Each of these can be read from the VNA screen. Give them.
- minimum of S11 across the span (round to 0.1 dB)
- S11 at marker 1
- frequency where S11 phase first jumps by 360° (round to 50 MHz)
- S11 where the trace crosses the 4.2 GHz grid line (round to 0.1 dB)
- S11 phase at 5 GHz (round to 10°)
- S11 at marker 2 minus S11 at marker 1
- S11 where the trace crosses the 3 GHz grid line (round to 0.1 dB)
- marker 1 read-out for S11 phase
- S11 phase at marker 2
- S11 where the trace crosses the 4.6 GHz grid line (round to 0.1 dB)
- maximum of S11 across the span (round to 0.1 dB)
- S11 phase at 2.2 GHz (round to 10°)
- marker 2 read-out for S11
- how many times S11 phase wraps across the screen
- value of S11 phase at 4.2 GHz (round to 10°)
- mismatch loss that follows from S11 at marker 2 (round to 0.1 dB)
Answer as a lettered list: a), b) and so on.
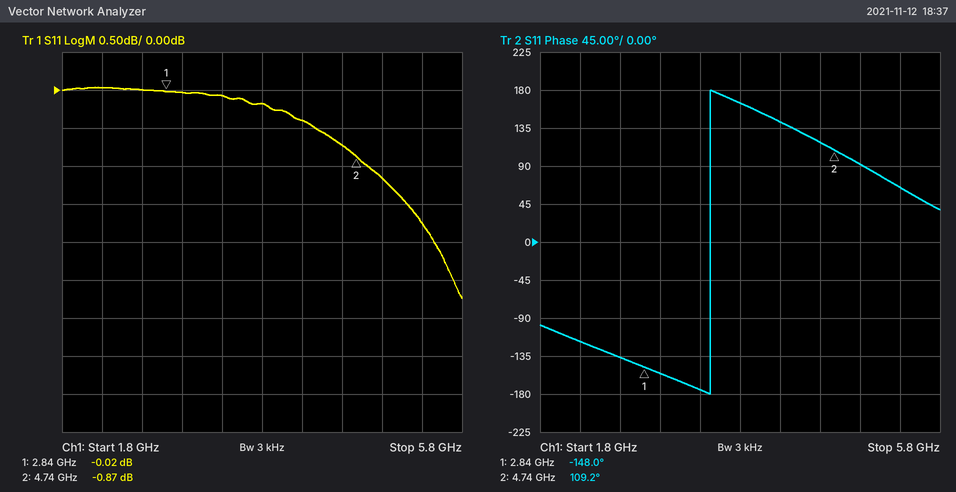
a) -2.7 dB
b) -0.02 dB
c) 3.50 GHz
d) -0.4 dB
e) 90°
f) -0.85 dB
g) 0.0 dB
h) -148.0°
i) 109.2°
j) -0.7 dB
k) 0.0 dB
l) -120°
m) -0.87 dB
n) 1
o) 140°
p) 7.4 dB
